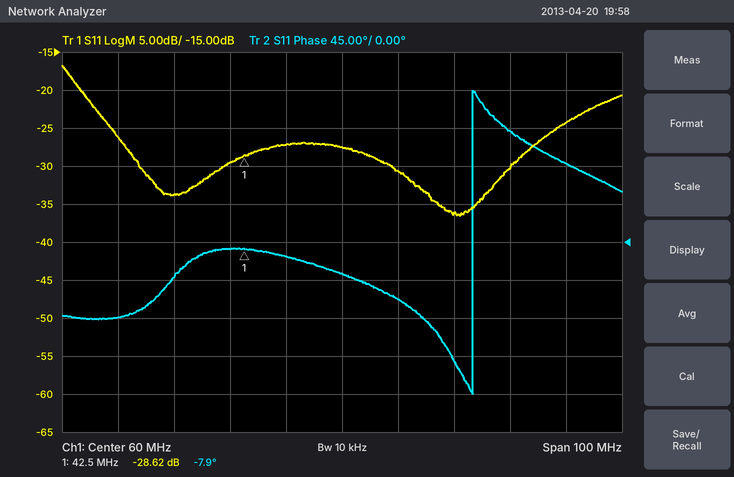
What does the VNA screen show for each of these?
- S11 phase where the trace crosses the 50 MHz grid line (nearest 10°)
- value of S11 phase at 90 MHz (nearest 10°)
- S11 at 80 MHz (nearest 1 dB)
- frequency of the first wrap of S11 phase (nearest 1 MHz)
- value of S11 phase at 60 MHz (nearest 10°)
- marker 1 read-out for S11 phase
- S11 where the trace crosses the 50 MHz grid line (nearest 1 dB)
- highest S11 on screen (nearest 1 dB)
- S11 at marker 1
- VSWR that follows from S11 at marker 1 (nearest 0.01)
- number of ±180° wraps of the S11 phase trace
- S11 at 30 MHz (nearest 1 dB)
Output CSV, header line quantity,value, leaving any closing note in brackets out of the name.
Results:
quantity,value
S11 phase where the trace crosses the 50 MHz grid line,-20°
value of S11 phase at 90 MHz,130°
S11 at 80 MHz,-36 dB
frequency of the first wrap of S11 phase,83 MHz
value of S11 phase at 60 MHz,-40°
marker 1 read-out for S11 phase,-7.9°
S11 where the trace crosses the 50 MHz grid line,-27 dB
highest S11 on screen,-17 dB
S11 at marker 1,-28.62 dB
VSWR that follows from S11 at marker 1,1.08
number of ±180° wraps of the S11 phase trace,1
S11 at 30 MHz,-34 dB
